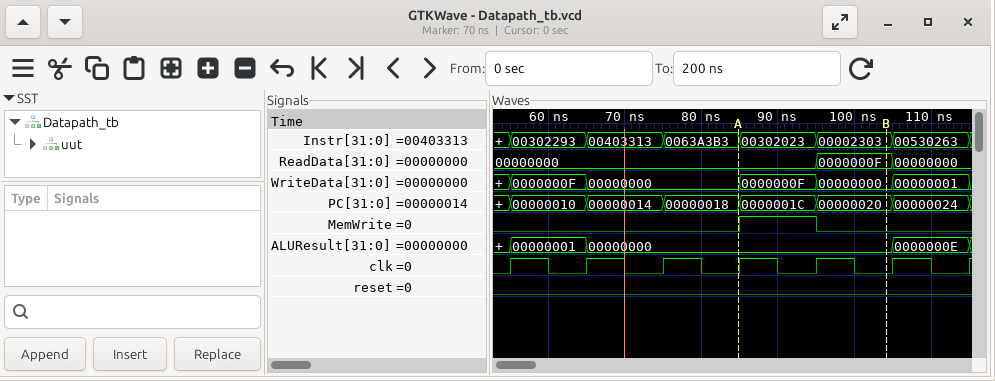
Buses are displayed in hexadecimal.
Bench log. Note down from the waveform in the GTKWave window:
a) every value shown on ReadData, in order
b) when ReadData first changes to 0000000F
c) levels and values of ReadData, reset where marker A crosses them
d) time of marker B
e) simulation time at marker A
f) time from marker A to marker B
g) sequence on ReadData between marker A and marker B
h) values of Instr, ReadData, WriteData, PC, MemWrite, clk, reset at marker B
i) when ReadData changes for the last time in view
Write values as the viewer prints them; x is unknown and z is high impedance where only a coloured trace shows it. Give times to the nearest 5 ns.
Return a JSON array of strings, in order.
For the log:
["00000000, 0000000F, 00000000", "95 ns", "ReadData=00000000, reset=0", "105 ns", "85 ns", "20 ns", "00000000, 0000000F", "Instr=00002303, ReadData=0000000F, WriteData=00000000, PC=00000020, MemWrite=0, clk=0, reset=0", "105 ns"]
